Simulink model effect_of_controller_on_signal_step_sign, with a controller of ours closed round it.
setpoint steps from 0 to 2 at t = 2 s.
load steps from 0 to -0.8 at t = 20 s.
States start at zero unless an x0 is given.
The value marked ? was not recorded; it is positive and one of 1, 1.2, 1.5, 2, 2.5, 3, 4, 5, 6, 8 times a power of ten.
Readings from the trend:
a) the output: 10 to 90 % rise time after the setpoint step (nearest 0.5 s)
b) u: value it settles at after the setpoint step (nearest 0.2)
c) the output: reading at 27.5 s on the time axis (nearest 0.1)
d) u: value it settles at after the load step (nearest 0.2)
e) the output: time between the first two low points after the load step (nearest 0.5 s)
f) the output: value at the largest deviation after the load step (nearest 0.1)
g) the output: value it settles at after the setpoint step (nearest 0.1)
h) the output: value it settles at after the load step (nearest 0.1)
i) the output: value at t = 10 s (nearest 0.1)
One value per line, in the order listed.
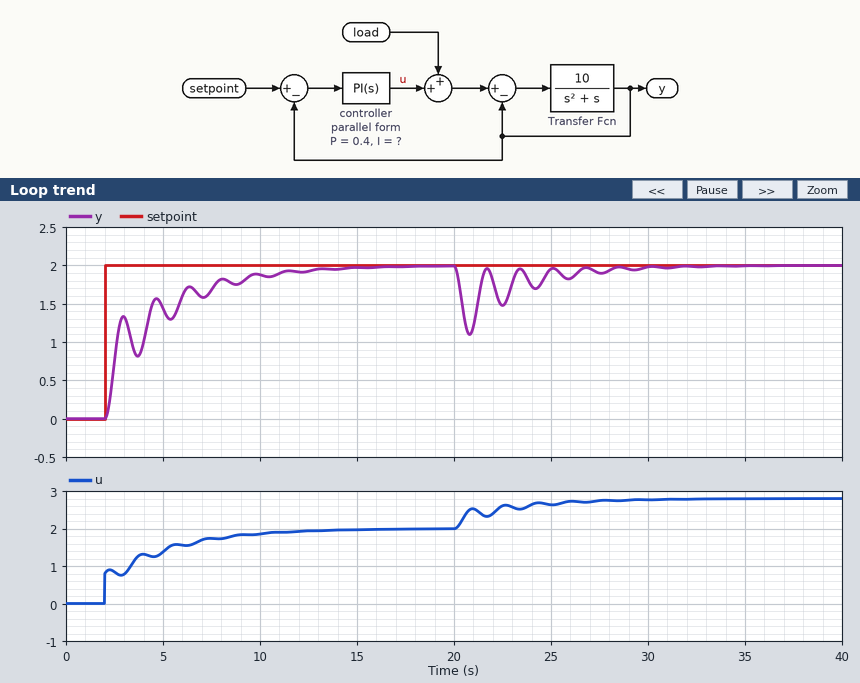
5.5 s
2.0
1.9
2.8
1.5 s
1.1
2.0
2.0
1.9
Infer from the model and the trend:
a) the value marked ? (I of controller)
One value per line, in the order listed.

0.4
